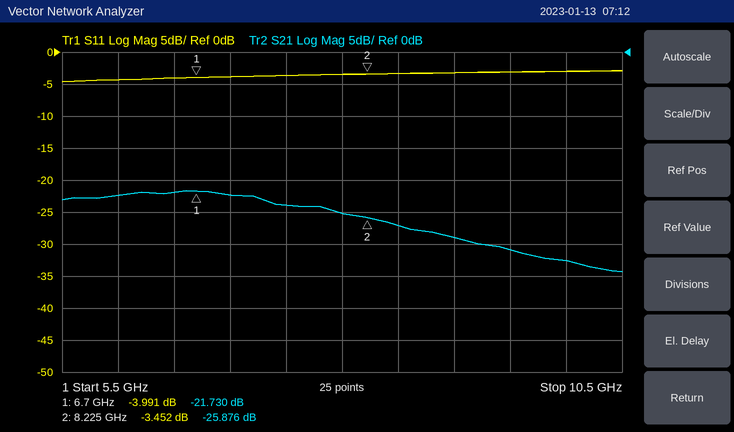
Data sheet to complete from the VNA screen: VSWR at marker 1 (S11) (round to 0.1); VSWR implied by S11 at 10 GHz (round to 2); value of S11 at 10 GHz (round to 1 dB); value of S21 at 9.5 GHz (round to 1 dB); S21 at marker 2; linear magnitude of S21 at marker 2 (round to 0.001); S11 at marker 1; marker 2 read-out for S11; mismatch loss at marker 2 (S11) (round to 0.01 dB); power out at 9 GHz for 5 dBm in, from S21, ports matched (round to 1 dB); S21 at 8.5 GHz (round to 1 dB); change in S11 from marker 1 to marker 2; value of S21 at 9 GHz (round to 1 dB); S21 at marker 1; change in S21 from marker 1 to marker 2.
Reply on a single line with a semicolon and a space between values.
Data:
4.4; 6; -3 dB; -31 dB; -25.876 dB; 0.051; -3.991 dB; -3.452 dB; 2.61 dB; -24 dBm; -27 dB; 0.539 dB; -29 dB; -21.730 dB; -4.146 dB
